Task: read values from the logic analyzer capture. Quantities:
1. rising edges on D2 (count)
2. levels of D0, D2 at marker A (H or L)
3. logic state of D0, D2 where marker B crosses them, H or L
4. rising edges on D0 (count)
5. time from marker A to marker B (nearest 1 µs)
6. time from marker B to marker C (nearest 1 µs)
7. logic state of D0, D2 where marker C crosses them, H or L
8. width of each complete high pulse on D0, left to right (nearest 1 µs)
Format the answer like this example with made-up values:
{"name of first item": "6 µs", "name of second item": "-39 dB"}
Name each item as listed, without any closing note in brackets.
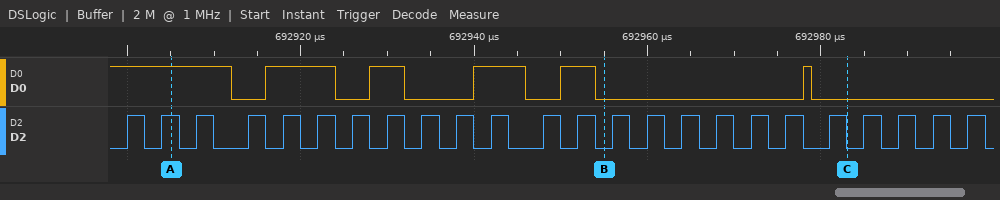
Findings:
{"rising edges on D2": "24", "levels of D0, D2 at marker A": "D0=H, D2=H", "logic state of D0, D2 where marker B crosses them, H or L": "D0=L, D2=L", "rising edges on D0": "5", "time from marker A to marker B": "50 µs", "time from marker B to marker C": "28 µs", "logic state of D0, D2 where marker C crosses them, H or L": "D0=L, D2=L", "width of each complete high pulse on D0, left to right": "8 µs, 4 µs, 6 µs, 4 µs, 1 µs"}
